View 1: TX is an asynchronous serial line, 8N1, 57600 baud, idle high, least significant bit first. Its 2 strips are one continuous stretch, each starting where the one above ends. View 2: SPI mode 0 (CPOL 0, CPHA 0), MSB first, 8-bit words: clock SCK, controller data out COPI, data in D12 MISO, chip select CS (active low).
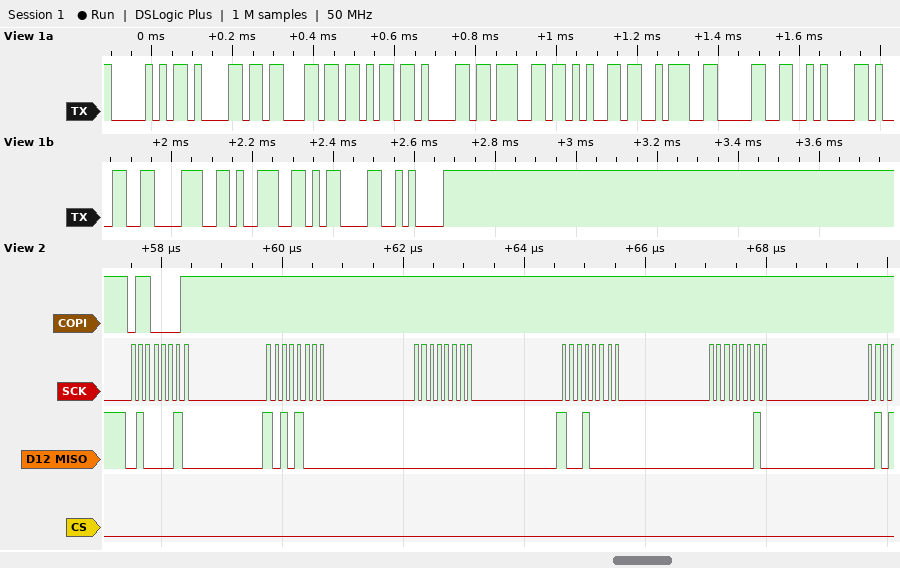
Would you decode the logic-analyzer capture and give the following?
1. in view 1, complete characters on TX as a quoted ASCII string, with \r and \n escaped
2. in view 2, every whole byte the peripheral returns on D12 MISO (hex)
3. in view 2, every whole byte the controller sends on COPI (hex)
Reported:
"Package:0\n189\r\n"
0x42 0xA8 0x00 0x90 0x02
0x61 0xFF 0xFF 0xFF 0xFF
